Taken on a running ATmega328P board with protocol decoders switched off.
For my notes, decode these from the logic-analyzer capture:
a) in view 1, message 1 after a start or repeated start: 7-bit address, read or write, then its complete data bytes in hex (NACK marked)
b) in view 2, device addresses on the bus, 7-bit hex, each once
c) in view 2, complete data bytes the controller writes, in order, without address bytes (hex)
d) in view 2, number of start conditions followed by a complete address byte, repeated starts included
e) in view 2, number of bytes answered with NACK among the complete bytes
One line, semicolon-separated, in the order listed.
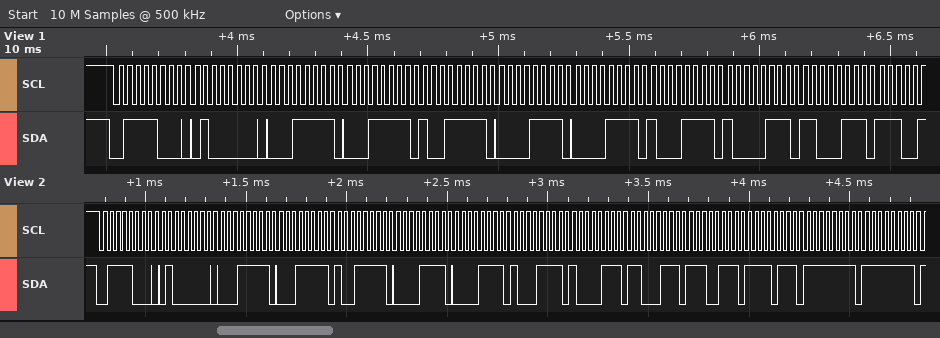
0x3C write: 40 1F 1F 9F 0F 0F 8F 87 C7; 0x3C; 40 1F 1F 9F 0F 0F 8F 87 C7 E7 F7 FF FF; 1; 0
